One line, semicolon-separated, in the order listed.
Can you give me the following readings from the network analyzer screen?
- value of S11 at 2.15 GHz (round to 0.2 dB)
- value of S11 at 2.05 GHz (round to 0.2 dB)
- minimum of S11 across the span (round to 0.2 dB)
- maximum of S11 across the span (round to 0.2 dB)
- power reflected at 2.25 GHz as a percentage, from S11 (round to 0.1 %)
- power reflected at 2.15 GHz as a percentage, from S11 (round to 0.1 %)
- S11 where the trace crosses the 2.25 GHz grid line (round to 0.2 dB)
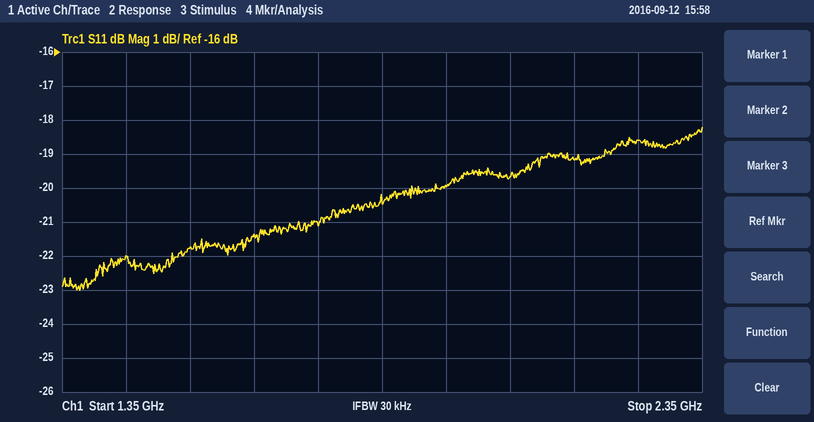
-19.2 dB; -19.6 dB; -23.0 dB; -18.2 dB; 1.4 %; 1.2 %; -18.6 dB
